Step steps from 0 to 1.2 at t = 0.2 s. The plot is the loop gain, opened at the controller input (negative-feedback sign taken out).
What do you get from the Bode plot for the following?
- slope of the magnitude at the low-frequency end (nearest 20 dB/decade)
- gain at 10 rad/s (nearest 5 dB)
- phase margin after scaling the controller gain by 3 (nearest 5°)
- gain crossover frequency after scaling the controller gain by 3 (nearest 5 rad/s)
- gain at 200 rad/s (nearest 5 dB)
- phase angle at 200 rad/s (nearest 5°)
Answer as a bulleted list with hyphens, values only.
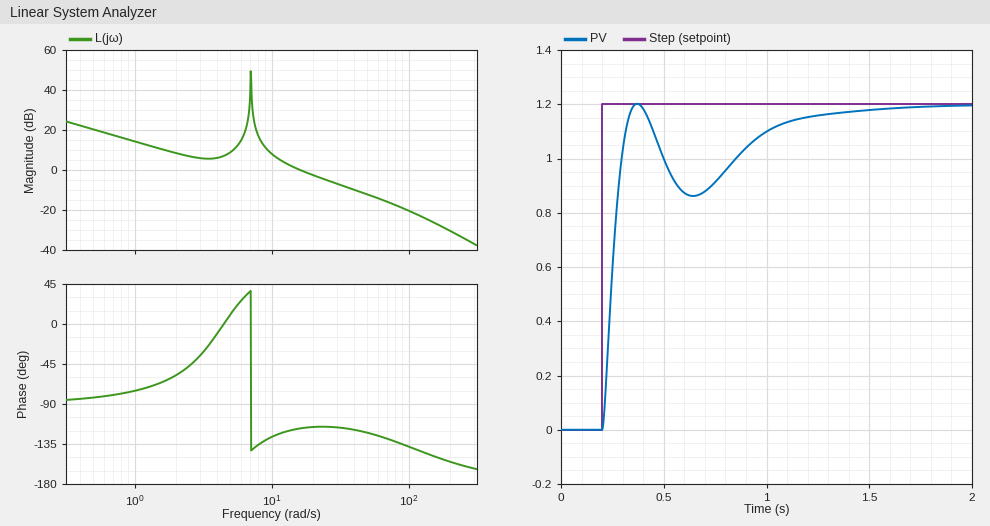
- -20 dB/decade
- 10 dB
- 60°
- 40 rad/s
- -30 dB
- -155°
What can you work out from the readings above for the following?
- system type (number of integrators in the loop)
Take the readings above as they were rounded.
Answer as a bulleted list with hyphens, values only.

- 1
